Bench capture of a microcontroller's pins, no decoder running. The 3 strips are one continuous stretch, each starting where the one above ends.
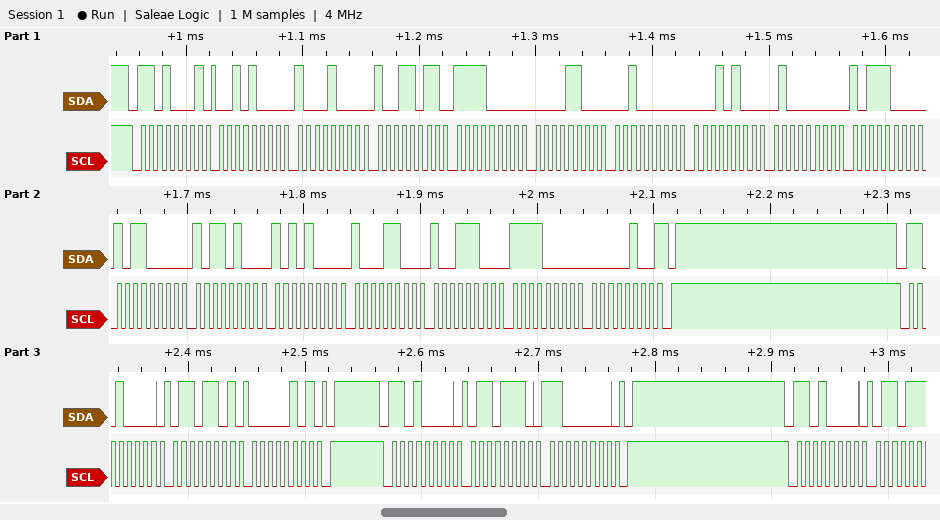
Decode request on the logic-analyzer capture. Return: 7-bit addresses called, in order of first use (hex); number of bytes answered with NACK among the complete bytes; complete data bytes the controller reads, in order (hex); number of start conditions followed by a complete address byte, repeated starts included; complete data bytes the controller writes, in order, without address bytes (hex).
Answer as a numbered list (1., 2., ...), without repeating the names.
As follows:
1. 0x68
2. 1
3. 28 88 9B F0 0C 20 14 40 B8 B0 B4 A8 8C 9C F0 04
4. 4
5. 6D 05 6E C0
